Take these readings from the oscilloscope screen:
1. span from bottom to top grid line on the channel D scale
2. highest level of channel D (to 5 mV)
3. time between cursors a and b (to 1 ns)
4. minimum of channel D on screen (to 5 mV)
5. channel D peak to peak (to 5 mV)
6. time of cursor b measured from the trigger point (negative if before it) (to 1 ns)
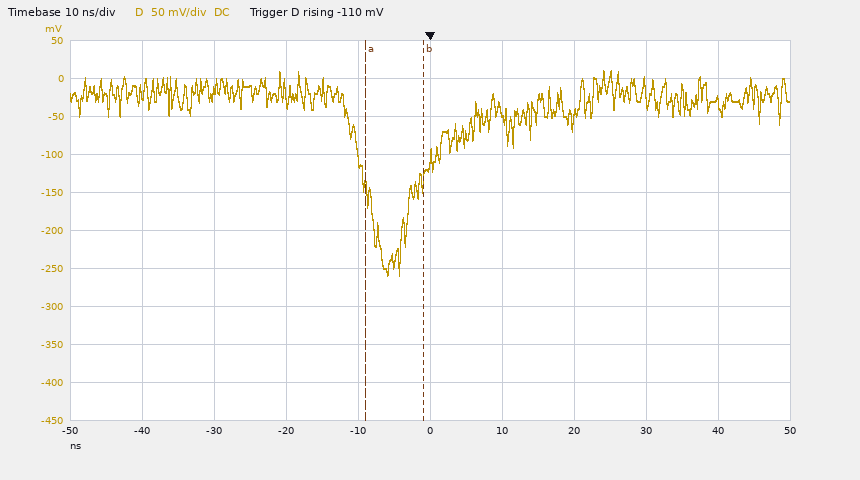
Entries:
500 mV
10 mV
8 ns
-260 mV
270 mV
-1 ns
